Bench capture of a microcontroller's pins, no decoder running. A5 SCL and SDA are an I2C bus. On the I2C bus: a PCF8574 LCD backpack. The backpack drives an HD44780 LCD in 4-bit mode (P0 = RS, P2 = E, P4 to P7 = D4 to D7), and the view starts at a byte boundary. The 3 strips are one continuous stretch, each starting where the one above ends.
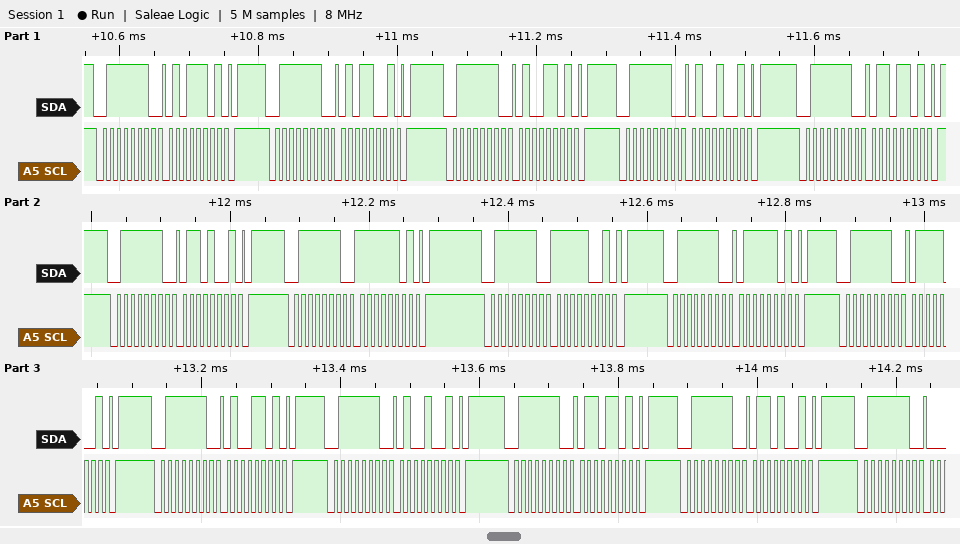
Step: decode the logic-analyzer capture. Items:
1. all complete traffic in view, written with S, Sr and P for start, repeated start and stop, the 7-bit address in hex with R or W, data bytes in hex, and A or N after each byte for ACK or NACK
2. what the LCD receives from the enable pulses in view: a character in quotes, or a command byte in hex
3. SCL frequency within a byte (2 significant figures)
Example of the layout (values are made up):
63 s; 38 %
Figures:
S 3FW A 5D A P S 3FW A 59 A P S 3FW A 4D A P S 3FW A 49 A P S 3FW A 6D A P S 3FW A 69 A P S 3FW A FD A P S 3FW A F9 A P S 3FW A 7D A P S 3FW A 79 A P S 3FW A 4D A P S 3FW A 49 A P S 3FW A 6D A P S 3FW A 69 A P S 3FW A; 'T' 'o' 't'; 100 kHz
